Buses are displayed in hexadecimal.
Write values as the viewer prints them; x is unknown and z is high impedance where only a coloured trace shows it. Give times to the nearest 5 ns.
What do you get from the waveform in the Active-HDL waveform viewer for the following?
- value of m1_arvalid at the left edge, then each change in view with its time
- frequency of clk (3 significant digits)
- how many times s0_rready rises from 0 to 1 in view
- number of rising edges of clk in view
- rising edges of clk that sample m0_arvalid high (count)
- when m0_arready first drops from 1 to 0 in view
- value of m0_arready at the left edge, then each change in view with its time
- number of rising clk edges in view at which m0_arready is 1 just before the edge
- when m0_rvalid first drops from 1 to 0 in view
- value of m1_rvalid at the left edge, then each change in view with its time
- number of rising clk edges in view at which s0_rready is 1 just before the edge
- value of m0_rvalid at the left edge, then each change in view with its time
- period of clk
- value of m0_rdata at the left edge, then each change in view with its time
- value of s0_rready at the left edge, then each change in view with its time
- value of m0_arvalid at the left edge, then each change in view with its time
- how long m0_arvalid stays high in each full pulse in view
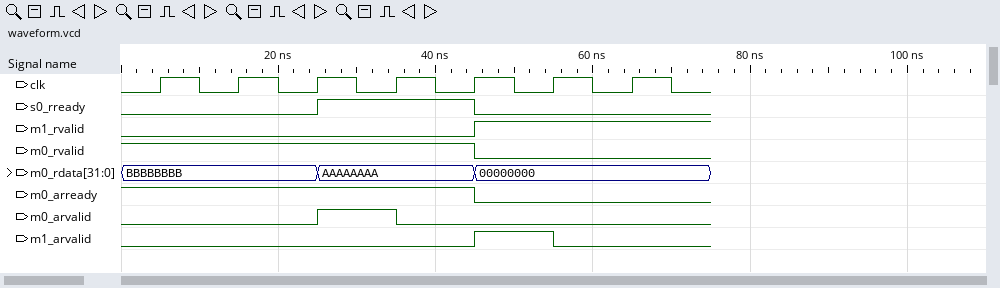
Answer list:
0, 1 at 45 ns, 0 at 55 ns
100 MHz
1
7
1
45 ns
1, 0 at 45 ns
5
45 ns
0, 1 at 45 ns
2
1, 0 at 45 ns
10 ns
BBBBBBBB, AAAAAAAA at 25 ns, 00000000 at 45 ns
0, 1 at 25 ns, 0 at 45 ns
0, 1 at 25 ns, 0 at 35 ns
10 ns
